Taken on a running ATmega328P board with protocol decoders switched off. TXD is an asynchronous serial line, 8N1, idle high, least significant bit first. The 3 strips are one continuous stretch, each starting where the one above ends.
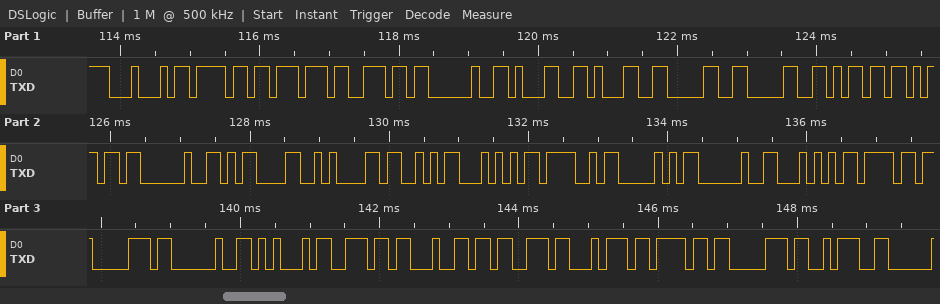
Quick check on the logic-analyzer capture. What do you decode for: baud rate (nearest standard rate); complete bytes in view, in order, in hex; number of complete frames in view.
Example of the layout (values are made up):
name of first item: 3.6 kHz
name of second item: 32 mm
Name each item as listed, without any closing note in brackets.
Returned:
baud rate: 9600 baud
complete bytes in view, in order, in hex: 44 6F 77 6E 20 31 31 30 30 6D 6D 20 0D 0A 53 54 4F 50 20 54 6F 70 20 45 6E 64 73 74 6F 70 3A
number of complete frames in view: 31
